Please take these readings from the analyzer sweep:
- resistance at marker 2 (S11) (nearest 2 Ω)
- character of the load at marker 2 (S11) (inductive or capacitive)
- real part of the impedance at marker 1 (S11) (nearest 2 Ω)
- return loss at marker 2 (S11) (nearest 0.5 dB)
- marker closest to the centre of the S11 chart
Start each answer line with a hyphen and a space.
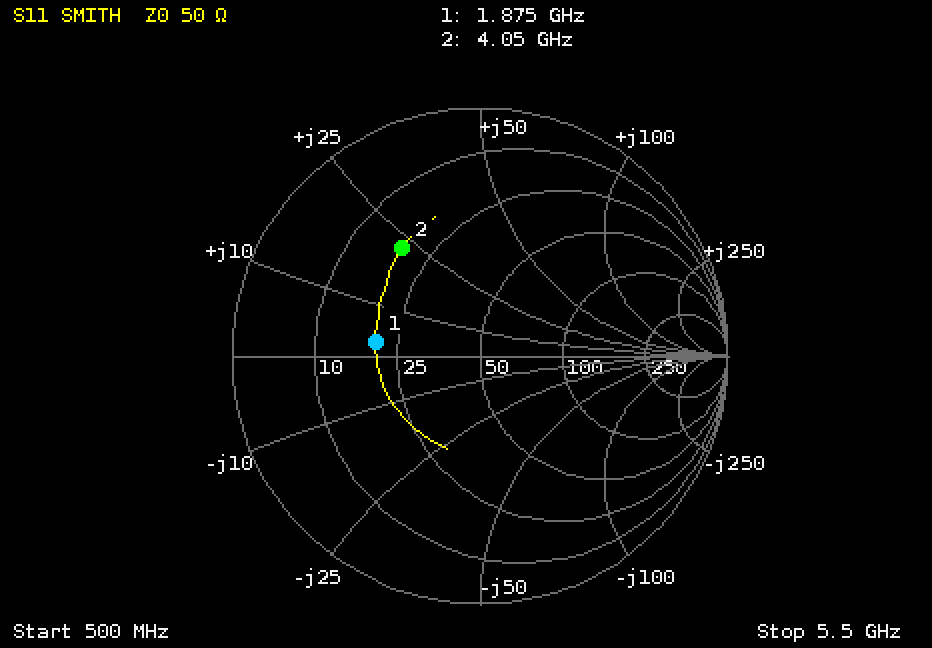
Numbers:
- 18 Ω
- inductive
- 20 Ω
- 5.5 dB
- marker 1
